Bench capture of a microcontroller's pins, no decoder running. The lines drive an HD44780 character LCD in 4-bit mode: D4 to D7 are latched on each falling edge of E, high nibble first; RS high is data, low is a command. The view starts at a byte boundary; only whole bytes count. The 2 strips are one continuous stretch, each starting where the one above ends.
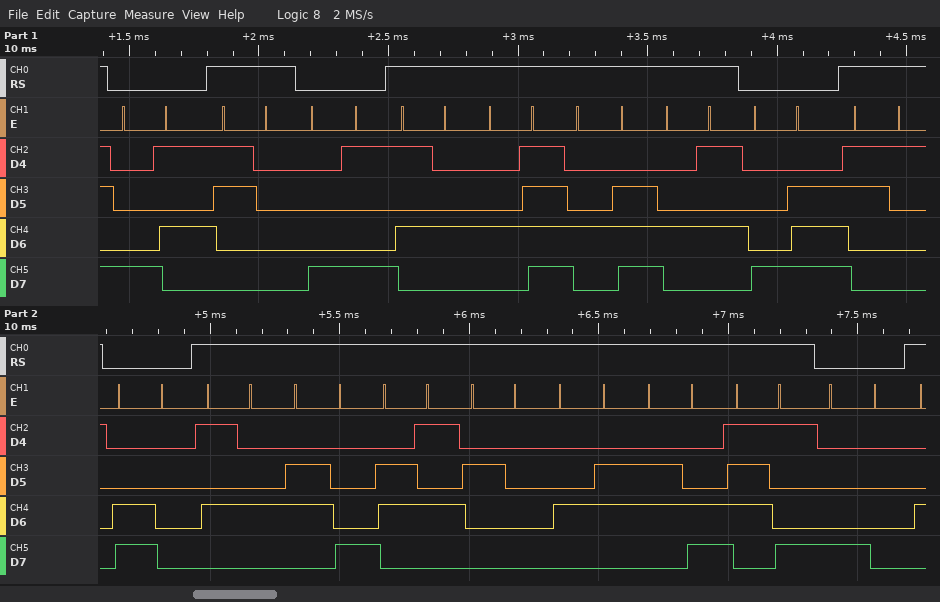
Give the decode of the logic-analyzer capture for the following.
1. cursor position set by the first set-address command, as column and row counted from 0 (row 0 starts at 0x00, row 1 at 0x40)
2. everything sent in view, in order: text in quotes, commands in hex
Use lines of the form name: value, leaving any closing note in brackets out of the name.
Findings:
cursor position set by the first set-address command, as column and row counted from 0: column 5, row 0
everything sent in view, in order: text in quotes, commands in hex: 0x85 "0" 0x89 "TONE" 0x8E "1" 0xC0 "The Fly" 0x80
